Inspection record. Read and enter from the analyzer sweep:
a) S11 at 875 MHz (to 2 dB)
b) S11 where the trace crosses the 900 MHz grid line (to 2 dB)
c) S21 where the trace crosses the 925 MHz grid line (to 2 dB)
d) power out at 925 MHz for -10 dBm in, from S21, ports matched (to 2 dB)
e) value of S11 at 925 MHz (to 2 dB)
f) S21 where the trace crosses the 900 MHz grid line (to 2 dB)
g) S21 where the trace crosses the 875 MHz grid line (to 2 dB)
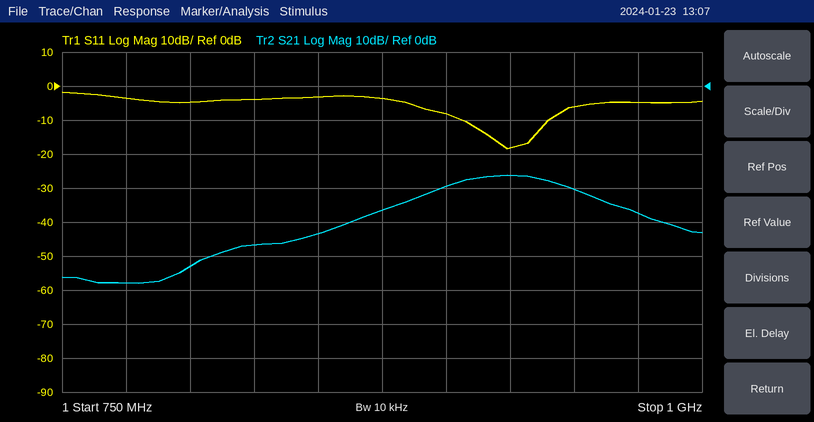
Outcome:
-4 dB
-8 dB
-26 dB
-36 dBm
-18 dB
-30 dB
-36 dB
